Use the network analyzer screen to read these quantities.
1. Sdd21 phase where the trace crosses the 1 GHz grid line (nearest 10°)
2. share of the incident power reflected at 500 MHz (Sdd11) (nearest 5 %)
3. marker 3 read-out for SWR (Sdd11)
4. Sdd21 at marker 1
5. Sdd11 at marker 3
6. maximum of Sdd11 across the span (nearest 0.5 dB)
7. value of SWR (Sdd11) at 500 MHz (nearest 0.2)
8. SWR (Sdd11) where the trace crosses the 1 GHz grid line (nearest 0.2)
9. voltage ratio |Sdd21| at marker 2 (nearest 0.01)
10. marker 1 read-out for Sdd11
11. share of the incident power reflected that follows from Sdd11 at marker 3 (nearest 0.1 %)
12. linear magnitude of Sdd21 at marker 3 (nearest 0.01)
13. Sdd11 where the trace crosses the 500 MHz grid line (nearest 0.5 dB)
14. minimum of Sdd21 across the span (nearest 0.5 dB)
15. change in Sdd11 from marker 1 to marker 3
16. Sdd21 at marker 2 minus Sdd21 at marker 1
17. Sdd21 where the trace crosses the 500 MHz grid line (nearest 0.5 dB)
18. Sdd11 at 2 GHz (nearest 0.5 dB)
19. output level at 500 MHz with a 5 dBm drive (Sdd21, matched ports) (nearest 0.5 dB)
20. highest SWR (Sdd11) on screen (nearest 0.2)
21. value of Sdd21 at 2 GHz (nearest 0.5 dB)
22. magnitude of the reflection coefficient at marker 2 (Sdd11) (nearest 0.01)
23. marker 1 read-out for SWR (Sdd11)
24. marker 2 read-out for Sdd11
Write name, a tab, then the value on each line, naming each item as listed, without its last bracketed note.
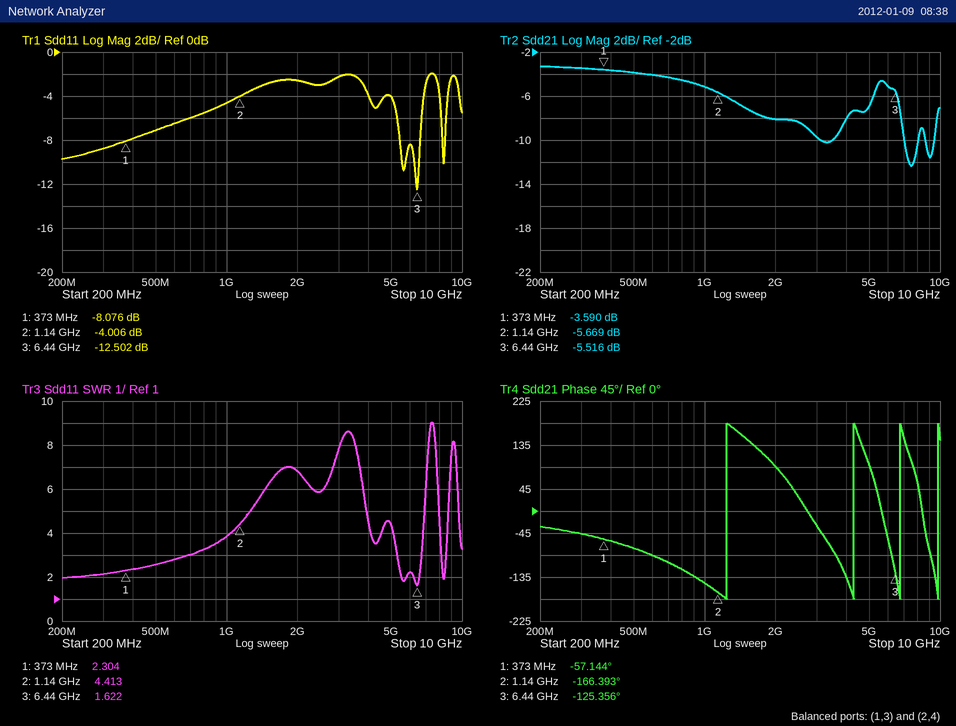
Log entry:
Sdd21 phase where the trace crosses the 1 GHz grid line	-150°
share of the incident power reflected at 500 MHz (Sdd11)	20 %
marker 3 read-out for SWR	1.622
Sdd21 at marker 1	-3.590 dB
Sdd11 at marker 3	-12.502 dB
maximum of Sdd11 across the span	-2.0 dB
value of SWR (Sdd11) at 500 MHz	2.6
SWR (Sdd11) where the trace crosses the 1 GHz grid line	3.8
voltage ratio |Sdd21| at marker 2	0.52
marker 1 read-out for Sdd11	-8.076 dB
share of the incident power reflected that follows from Sdd11 at marker 3	5.6 %
linear magnitude of Sdd21 at marker 3	0.53
Sdd11 where the trace crosses the 500 MHz grid line	-7.0 dB
minimum of Sdd21 across the span	-12.5 dB
change in Sdd11 from marker 1 to marker 3	-4.426 dB
Sdd21 at marker 2 minus Sdd21 at marker 1	-2.079 dB
Sdd21 where the trace crosses the 500 MHz grid line	-4.0 dB
Sdd11 at 2 GHz	-2.5 dB
output level at 500 MHz with a 5 dBm drive (Sdd21, matched ports)	1.0 dBm
highest SWR (Sdd11) on screen	9.0
value of Sdd21 at 2 GHz	-8.0 dB
magnitude of the reflection coefficient at marker 2 (Sdd11)	0.63
marker 1 read-out for SWR	2.304
marker 2 read-out for Sdd11	-4.006 dB
